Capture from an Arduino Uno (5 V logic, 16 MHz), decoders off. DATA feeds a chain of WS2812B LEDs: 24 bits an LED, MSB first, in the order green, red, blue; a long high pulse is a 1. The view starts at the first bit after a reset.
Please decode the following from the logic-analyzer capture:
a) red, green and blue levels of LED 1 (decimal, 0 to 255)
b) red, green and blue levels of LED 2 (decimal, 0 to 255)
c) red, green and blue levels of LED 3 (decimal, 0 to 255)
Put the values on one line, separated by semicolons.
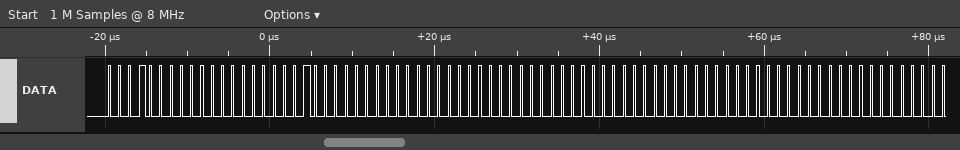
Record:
0, 16, 16; 0, 0, 0; 0, 0, 0
